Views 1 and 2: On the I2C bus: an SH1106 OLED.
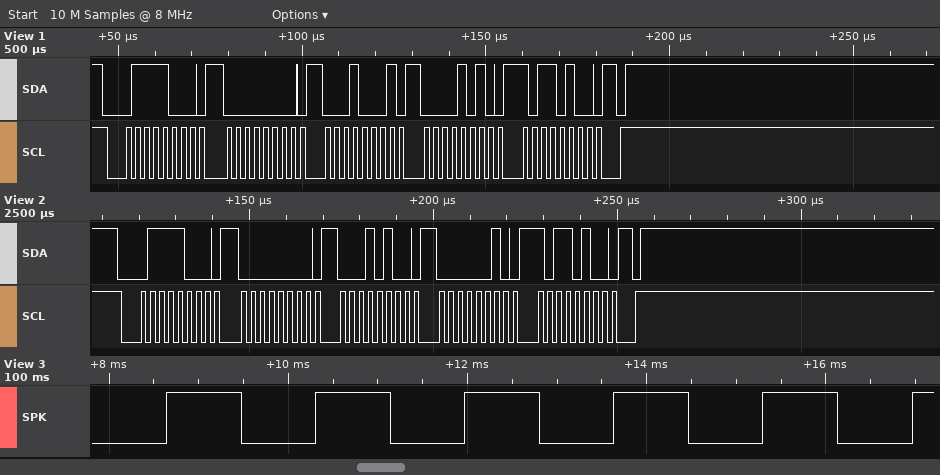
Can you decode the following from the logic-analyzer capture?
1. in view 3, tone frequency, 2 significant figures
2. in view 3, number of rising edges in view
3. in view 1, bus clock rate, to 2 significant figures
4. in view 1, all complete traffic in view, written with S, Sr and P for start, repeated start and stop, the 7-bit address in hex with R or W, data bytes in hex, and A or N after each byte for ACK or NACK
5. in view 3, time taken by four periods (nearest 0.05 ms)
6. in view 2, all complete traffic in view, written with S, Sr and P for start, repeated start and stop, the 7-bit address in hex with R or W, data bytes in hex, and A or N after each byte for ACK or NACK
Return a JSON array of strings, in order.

["600 Hz", "6", "400 kHz", "S 3CW A 00 A 11 A 0A A B4 A P", "6.65 ms", "S 3CW A 00 A 14 A 02 A B4 A P"]
